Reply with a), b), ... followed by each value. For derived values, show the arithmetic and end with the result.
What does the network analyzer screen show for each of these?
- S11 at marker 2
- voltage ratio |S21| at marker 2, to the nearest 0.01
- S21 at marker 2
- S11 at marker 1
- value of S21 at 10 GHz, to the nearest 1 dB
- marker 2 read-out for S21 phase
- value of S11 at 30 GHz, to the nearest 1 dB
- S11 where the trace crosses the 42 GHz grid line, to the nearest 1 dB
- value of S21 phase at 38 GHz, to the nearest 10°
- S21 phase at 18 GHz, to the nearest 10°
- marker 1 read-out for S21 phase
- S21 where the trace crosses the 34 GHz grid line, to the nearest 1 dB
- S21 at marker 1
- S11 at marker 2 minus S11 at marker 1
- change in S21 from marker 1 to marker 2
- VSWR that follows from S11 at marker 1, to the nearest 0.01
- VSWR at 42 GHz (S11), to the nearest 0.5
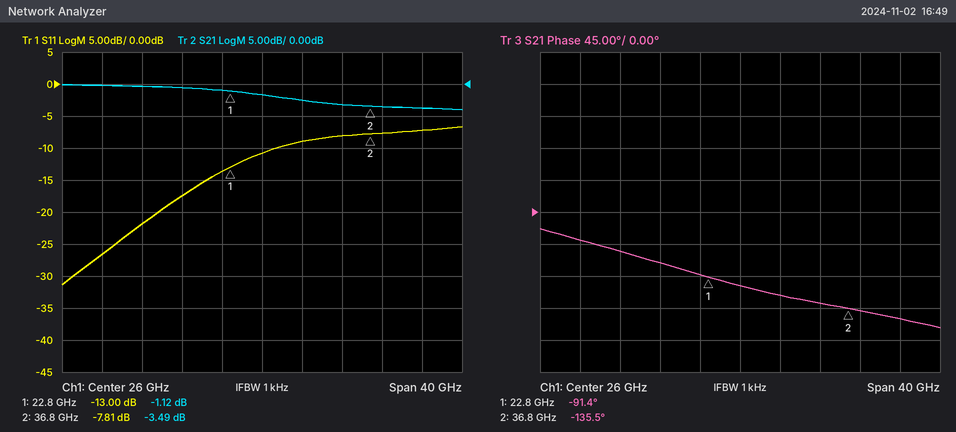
a) -7.81 dB
b) 10^(-3.49/20) ≈ 0.67
c) -3.49 dB
d) -13.00 dB
e) 0 dB
f) -135.5°
g) -9 dB
h) -7 dB
i) -140°
j) -70°
k) -91.4°
l) -3 dB
m) -1.12 dB
n) -7.81 − (-13) = 5.19 dB
o) -3.49 − (-1.12) = -2.37 dB
p) (1 + 0.2239)/(1 − 0.2239) ≈ 1.58
q) |Γ| = 10^(-7/20) = 0.4467; VSWR = (1 + 0.4467)/(1 − 0.4467) ≈ 2.61, so 2.5 to the nearest 0.5
